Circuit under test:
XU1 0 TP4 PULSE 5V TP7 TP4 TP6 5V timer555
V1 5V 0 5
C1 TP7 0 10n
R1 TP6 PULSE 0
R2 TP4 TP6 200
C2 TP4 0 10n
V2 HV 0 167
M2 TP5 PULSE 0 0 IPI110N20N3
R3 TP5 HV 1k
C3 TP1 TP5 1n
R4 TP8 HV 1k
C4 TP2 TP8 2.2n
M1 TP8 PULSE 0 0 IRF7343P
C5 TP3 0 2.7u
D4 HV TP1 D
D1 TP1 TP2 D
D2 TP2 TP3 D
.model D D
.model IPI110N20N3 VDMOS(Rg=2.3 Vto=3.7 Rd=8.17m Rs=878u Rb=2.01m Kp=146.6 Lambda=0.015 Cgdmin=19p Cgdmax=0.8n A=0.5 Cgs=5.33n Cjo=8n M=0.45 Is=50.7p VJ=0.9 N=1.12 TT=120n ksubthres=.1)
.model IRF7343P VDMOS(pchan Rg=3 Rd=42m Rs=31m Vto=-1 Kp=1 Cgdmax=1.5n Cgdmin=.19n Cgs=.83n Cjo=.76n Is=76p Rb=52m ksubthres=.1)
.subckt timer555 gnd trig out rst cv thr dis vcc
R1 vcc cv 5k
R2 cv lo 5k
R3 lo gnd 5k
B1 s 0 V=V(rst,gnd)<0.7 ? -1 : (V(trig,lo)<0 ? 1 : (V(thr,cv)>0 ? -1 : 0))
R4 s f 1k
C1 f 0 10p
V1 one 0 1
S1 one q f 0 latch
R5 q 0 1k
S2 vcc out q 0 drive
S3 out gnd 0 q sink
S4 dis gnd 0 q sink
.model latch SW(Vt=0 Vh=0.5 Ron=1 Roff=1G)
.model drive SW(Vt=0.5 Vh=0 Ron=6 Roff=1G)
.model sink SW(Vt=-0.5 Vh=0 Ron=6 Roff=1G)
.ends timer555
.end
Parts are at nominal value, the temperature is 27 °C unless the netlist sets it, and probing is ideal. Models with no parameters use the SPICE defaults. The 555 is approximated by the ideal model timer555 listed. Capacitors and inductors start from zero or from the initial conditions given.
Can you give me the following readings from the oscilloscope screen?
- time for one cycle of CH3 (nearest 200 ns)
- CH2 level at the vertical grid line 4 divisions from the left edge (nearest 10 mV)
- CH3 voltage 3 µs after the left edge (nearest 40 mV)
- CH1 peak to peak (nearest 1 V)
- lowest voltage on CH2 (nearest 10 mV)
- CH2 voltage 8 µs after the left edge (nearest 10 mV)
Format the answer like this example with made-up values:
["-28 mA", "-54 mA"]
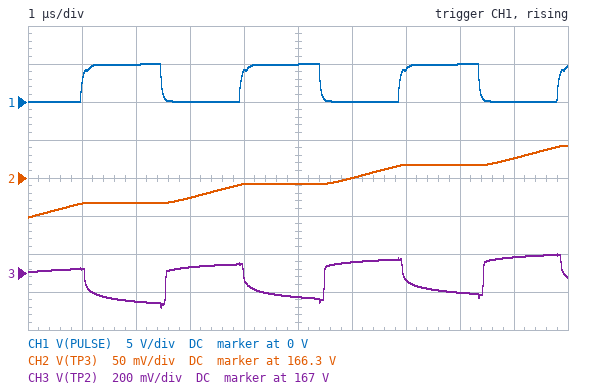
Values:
["3.0 µs", "166.29 V", "167.04 V", "5 V", "166.25 V", "166.32 V"]
